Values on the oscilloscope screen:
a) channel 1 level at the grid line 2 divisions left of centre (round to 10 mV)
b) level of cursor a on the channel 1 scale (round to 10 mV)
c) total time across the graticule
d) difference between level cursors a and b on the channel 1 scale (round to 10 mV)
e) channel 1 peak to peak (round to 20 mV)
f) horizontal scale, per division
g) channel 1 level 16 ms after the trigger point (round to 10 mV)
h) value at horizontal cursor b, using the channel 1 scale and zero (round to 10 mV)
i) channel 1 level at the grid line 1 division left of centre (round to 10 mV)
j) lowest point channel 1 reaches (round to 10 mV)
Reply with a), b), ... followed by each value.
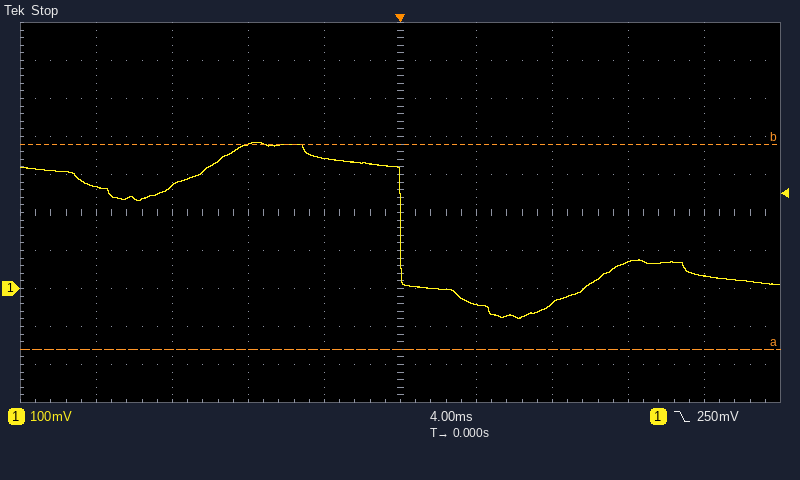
a) 380 mV
b) -160 mV
c) 40 ms
d) 540 mV
e) 460 mV
f) 4 ms
g) 30 mV
h) 380 mV
i) 340 mV
j) -80 mV
